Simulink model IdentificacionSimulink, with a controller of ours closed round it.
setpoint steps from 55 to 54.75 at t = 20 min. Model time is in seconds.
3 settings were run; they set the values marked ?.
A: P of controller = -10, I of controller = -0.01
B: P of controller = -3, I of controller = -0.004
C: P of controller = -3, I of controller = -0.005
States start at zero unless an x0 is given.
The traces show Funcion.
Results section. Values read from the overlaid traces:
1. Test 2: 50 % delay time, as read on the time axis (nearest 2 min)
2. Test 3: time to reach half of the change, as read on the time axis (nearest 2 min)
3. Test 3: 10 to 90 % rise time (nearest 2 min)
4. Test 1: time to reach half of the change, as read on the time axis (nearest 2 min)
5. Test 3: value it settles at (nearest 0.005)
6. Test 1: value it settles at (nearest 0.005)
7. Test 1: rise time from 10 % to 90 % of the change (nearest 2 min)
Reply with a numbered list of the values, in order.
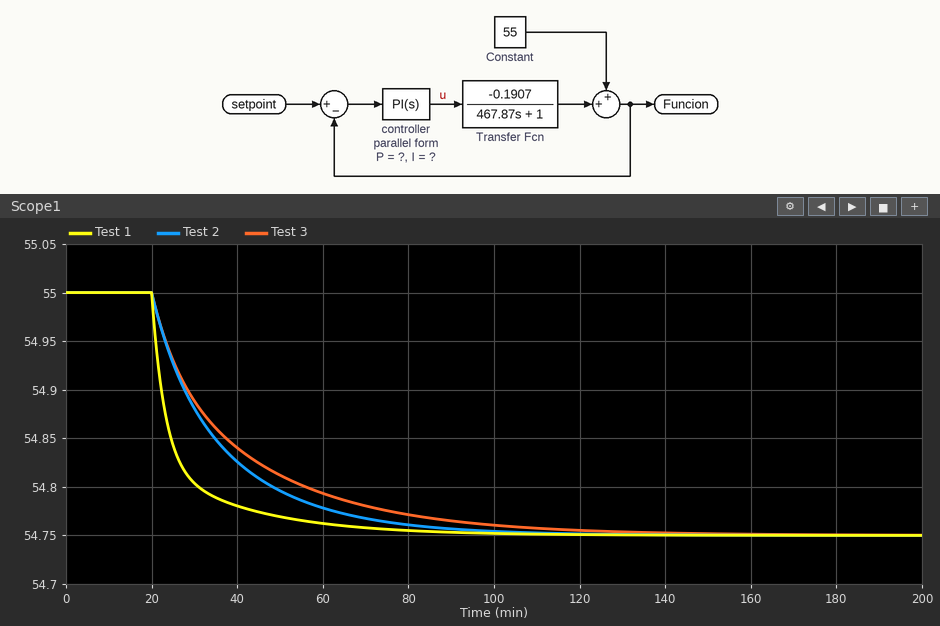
1. 30 min
2. 32 min
3. 54 min
4. 24 min
5. 54.750
6. 54.750
7. 24 min
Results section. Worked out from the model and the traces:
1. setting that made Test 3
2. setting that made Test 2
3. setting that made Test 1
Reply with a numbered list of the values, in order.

1. B
2. C
3. A
